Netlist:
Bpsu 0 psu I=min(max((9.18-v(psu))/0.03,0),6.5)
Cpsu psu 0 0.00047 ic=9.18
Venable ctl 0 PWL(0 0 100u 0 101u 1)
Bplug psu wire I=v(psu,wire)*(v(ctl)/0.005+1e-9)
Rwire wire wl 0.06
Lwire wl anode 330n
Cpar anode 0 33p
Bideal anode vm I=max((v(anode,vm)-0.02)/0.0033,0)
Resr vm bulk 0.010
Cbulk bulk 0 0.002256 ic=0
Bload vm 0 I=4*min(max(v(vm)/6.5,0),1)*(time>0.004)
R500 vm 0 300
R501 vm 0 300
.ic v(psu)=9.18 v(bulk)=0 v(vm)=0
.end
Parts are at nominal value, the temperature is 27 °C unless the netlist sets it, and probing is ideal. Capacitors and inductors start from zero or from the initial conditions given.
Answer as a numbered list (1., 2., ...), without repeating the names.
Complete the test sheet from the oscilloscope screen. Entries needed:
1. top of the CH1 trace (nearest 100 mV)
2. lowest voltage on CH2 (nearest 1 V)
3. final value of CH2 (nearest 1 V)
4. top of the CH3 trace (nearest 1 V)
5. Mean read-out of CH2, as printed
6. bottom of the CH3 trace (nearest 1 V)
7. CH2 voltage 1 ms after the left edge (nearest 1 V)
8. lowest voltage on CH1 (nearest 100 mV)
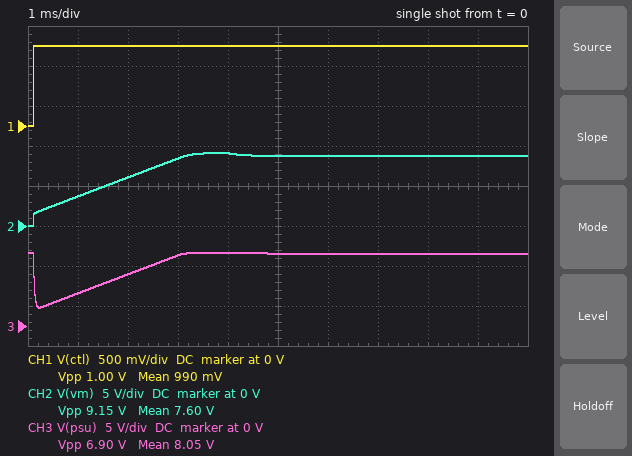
1. 1.0 V
2. 0 V
3. 9 V
4. 9 V
5. 7.60 V
6. 2 V
7. 4 V
8. 0 V
